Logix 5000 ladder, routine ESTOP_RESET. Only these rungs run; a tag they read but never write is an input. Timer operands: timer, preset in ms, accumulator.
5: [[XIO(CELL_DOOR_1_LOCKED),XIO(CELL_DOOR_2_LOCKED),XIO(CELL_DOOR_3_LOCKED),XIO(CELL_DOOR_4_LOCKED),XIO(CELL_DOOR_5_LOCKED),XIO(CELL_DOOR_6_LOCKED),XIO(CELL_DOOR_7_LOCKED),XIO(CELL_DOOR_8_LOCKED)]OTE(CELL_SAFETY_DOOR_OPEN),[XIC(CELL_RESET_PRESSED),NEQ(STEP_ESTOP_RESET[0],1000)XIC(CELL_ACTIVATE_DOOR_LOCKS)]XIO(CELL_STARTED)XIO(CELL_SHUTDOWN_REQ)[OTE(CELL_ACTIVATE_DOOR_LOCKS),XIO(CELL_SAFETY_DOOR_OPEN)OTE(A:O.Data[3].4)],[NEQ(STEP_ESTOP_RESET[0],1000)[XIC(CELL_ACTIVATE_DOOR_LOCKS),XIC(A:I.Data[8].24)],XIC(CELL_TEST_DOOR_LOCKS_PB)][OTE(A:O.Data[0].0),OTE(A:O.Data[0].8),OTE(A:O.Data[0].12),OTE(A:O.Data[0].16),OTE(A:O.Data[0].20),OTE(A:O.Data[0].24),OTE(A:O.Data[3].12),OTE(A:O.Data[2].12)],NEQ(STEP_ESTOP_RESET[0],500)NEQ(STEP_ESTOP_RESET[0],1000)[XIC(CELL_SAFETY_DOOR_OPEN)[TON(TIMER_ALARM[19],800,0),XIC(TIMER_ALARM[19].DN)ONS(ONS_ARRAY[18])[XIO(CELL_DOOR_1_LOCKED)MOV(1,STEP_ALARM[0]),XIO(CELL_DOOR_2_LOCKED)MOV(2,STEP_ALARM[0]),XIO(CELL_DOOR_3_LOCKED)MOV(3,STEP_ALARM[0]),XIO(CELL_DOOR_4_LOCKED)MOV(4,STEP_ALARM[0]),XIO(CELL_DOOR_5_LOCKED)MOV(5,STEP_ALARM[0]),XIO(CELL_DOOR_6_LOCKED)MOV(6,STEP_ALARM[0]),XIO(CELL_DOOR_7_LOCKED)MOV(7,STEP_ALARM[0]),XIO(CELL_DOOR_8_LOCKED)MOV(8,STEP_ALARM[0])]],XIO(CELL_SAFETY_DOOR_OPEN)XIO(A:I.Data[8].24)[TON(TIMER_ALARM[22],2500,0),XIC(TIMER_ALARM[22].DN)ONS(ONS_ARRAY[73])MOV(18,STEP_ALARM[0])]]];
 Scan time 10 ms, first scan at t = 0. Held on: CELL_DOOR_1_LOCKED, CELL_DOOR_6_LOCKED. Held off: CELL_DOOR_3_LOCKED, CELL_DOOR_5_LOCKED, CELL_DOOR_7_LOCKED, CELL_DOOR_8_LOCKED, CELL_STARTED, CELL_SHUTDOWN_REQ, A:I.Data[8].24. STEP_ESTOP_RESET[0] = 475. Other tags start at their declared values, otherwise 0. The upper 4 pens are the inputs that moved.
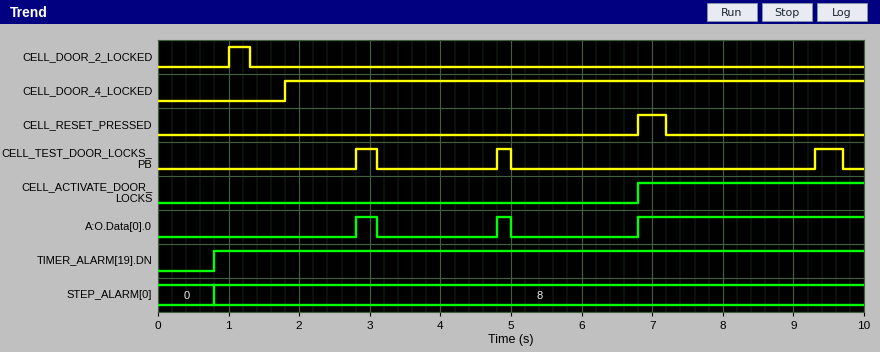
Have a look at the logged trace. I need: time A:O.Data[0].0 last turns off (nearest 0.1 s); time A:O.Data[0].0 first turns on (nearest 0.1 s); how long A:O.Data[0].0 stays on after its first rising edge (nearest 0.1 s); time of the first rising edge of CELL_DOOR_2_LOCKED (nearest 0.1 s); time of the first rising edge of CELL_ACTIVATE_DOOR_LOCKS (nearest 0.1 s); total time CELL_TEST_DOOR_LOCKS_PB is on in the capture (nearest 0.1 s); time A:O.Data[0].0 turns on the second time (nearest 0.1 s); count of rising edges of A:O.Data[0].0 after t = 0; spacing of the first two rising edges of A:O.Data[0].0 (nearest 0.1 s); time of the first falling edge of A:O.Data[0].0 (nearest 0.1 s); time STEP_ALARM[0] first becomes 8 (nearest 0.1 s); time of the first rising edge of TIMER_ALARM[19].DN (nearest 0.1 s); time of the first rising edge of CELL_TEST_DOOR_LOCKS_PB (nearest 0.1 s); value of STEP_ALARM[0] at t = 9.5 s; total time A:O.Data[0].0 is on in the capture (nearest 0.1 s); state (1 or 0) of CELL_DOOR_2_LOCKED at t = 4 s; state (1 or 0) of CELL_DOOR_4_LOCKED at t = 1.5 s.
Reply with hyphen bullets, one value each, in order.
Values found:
- 5.0 s
- 2.8 s
- 0.3 s
- 1.0 s
- 6.8 s
- 0.9 s
- 4.8 s
- 3
- 2.0 s
- 3.1 s
- 0.8 s
- 0.8 s
- 2.8 s
- 8
- 3.7 s
- 0
- 0
